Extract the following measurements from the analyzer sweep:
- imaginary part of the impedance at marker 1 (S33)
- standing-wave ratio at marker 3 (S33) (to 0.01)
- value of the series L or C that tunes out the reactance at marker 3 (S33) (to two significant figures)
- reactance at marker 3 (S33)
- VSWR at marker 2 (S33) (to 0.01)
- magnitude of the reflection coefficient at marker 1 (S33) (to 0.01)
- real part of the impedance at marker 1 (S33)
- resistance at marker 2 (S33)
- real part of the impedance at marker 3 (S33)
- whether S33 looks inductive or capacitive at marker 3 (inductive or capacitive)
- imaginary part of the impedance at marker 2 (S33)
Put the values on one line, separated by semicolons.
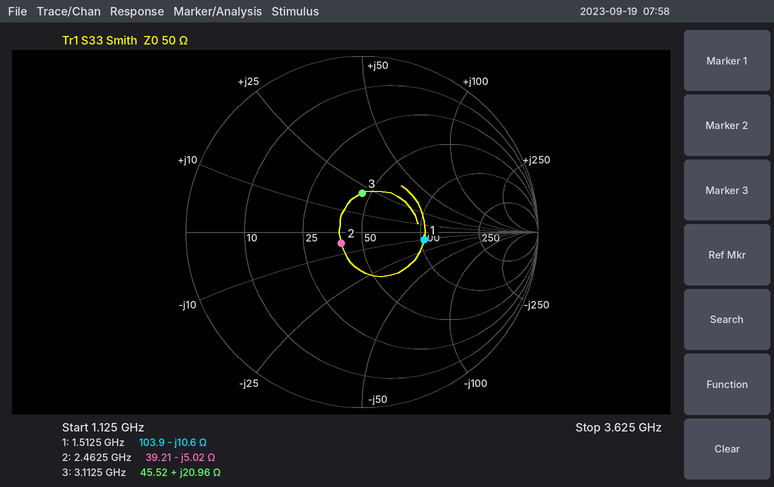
-10.6 Ω; 1.56; 2.4 pF; +20.96 Ω; 1.31; 0.36; 103.9 Ω; 39.21 Ω; 45.52 Ω; inductive; -5.02 Ω
